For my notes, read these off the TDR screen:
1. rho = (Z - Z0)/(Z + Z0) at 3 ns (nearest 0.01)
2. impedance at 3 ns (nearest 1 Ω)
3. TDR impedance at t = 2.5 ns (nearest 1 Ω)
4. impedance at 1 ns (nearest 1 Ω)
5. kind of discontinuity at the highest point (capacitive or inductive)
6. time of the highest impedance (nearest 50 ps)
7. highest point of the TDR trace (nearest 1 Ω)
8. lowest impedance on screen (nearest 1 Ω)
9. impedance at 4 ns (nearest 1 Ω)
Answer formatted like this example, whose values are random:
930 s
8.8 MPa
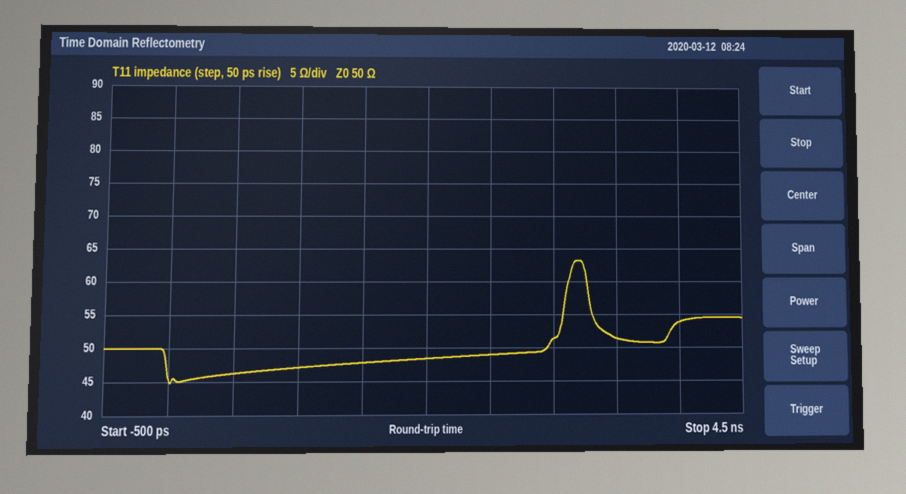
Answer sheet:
+0.01
51 Ω
49 Ω
47 Ω
inductive
3.20 ns
63 Ω
45 Ω
54 Ω
